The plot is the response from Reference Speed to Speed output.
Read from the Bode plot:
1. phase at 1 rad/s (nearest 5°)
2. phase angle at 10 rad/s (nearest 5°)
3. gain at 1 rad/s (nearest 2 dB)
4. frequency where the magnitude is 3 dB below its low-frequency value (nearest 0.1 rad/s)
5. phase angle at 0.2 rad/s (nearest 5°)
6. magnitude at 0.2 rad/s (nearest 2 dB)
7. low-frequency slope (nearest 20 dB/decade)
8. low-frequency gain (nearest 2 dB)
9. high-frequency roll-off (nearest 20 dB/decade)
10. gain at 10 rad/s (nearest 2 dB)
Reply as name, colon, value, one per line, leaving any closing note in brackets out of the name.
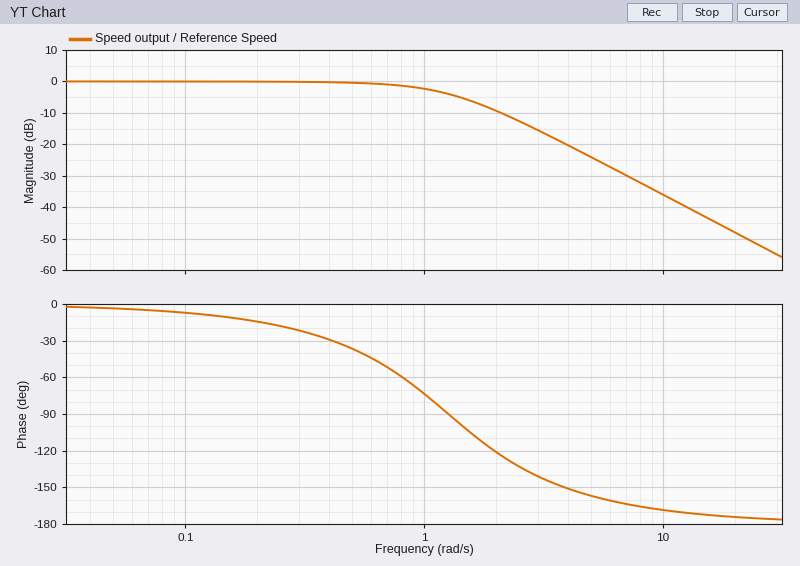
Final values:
phase at 1 rad/s: -75°
phase angle at 10 rad/s: -170°
gain at 1 rad/s: -2 dB
frequency where the magnitude is 3 dB below its low-frequency value: 1.1 rad/s
phase angle at 0.2 rad/s: -15°
magnitude at 0.2 rad/s: 0 dB
low-frequency slope: 0 dB/decade
low-frequency gain: 0 dB
high-frequency roll-off: -40 dB/decade
gain at 10 rad/s: -36 dB
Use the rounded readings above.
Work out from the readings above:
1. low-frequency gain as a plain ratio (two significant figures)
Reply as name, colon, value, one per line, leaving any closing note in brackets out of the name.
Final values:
low-frequency gain as a plain ratio: 1.0
